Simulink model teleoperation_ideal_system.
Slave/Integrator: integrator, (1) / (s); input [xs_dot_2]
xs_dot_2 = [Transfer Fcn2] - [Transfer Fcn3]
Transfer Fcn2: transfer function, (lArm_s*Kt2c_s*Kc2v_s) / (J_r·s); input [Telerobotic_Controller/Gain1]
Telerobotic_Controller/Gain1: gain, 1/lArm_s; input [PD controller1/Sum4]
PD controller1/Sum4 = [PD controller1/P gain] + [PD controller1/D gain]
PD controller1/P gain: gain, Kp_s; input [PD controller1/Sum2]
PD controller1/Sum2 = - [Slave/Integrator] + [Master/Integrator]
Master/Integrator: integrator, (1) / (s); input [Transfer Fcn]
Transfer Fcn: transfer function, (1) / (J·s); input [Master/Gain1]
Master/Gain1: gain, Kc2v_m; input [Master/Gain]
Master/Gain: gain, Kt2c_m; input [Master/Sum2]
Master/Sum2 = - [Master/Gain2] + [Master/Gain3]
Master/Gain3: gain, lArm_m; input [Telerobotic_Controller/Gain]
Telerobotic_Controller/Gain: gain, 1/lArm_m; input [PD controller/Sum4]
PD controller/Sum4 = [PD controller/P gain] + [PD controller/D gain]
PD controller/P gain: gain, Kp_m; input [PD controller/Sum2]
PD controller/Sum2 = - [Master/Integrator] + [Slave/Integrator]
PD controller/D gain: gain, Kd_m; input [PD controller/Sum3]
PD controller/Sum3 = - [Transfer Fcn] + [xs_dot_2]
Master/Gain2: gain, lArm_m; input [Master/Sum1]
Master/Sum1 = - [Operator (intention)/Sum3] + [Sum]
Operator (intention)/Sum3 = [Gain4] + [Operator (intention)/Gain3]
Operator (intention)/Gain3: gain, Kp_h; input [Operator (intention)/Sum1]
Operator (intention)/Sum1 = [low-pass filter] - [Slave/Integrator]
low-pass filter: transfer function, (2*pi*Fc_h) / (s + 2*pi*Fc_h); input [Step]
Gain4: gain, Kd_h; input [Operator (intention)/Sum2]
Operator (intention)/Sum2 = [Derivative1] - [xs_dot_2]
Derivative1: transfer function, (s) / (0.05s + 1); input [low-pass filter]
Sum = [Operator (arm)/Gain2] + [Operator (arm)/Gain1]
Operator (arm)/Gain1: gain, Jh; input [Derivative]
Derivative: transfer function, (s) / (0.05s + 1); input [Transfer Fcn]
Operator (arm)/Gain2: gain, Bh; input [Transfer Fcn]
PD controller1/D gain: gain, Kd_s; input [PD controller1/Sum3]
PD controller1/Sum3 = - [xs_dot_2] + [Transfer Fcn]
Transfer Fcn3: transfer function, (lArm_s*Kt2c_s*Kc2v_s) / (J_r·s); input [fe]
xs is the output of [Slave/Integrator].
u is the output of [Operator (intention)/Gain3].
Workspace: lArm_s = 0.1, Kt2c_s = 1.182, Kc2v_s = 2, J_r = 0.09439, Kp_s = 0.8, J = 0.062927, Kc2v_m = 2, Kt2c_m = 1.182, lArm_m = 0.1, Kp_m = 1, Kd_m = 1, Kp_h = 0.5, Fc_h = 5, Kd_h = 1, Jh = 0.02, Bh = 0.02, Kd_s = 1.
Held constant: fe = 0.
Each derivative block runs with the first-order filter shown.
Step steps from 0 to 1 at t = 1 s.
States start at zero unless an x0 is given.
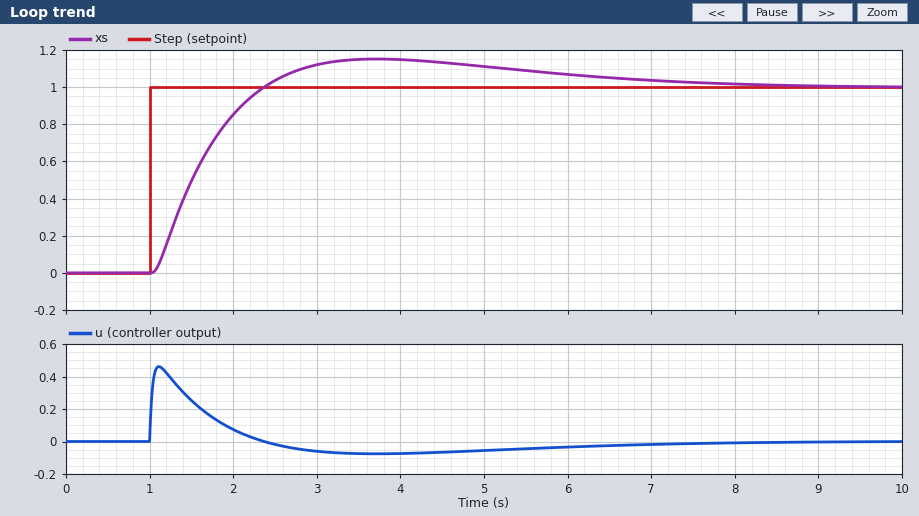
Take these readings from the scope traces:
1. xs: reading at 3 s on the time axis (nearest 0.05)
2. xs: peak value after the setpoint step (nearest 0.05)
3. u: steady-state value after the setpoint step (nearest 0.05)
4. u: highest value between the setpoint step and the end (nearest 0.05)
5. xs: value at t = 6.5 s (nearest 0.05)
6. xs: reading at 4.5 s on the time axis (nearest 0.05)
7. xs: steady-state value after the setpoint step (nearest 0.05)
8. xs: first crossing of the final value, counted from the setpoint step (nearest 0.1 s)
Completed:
1.10
1.15
0.00
0.45
1.05
1.15
1.00
1.4 s
